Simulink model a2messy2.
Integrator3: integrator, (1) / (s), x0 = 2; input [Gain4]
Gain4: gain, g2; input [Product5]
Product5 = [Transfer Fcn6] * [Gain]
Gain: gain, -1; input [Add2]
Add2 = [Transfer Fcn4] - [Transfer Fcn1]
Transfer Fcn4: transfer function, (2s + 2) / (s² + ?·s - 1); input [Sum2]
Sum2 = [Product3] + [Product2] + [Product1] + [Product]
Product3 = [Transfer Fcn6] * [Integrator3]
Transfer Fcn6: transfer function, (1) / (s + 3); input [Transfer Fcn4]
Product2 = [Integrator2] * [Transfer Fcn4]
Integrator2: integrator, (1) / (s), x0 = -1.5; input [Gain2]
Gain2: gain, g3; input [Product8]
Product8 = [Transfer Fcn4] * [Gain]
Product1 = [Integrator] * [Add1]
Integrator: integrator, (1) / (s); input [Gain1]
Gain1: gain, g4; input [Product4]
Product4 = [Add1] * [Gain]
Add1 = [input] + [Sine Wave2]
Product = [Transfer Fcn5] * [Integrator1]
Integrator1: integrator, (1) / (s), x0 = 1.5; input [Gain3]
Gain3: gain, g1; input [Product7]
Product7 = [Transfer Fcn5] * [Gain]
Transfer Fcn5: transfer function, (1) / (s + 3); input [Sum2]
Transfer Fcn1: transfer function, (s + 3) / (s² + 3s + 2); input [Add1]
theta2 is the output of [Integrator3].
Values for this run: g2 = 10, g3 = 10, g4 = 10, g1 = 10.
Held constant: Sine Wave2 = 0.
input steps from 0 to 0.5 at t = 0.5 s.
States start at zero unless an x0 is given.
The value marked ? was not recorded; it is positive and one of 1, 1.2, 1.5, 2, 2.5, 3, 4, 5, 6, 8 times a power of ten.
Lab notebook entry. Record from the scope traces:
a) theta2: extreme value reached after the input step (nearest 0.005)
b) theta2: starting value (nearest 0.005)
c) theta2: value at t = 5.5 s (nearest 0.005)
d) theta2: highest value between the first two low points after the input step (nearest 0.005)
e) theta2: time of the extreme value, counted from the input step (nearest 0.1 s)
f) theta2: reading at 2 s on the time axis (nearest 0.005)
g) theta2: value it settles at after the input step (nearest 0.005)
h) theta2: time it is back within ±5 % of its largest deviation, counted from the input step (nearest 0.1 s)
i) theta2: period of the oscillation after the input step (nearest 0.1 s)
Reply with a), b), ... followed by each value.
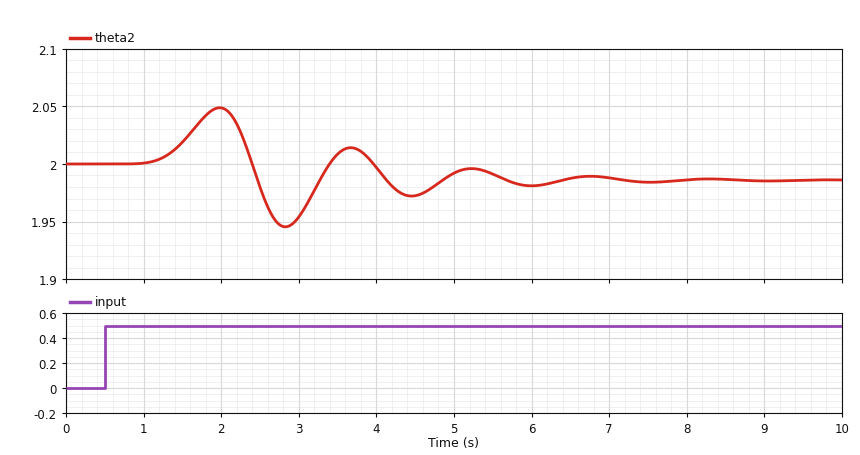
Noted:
a) 1.945
b) 2.000
c) 1.990
d) 2.015
e) 2.3 s
f) 2.050
g) 1.985
h) 6.4 s
i) 1.6 s
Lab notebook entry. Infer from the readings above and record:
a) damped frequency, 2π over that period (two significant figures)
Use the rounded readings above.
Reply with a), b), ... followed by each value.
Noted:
a) 3.9 rad/s
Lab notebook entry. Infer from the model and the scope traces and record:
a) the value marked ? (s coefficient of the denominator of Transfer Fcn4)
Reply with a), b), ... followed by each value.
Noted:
a) 1
